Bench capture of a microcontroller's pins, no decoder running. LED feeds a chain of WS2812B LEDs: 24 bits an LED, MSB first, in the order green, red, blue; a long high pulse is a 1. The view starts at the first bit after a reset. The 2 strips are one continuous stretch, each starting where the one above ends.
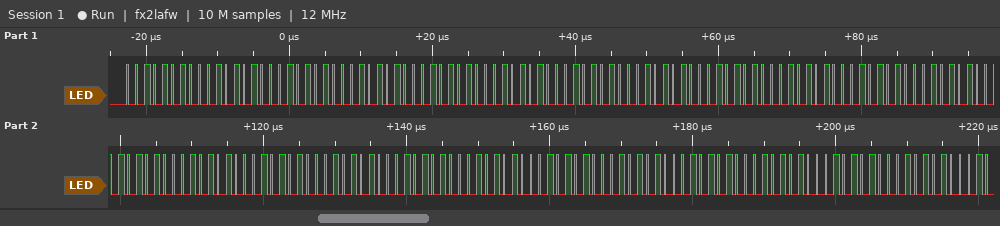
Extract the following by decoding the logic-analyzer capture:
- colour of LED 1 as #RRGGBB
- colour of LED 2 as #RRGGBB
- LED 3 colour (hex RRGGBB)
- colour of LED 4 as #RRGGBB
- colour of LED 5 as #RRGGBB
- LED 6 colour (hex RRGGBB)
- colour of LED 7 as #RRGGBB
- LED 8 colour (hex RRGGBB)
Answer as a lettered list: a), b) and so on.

a) #2A2A2A
b) #2A2A2A
c) #2A2A2A
d) #2A2A2A
e) #2A2A2A
f) #2A2A2A
g) #2A2A2A
h) #2A2A2A
